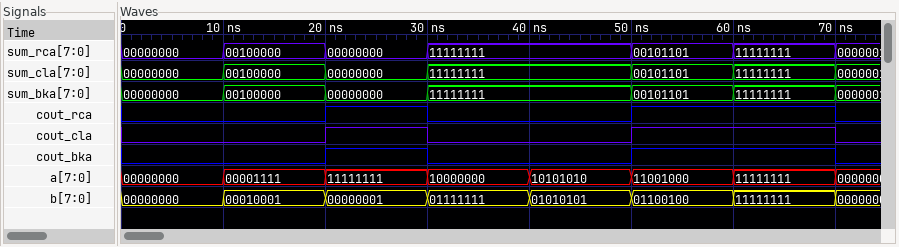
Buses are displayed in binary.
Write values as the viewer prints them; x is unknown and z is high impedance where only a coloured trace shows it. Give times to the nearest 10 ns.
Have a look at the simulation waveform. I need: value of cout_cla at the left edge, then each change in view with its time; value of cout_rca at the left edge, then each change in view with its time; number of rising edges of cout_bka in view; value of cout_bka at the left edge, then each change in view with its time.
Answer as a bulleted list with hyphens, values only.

- 0, 1 at 20 ns, 0 at 30 ns, 1 at 50 ns, 0 at 70 ns
- 0, 1 at 20 ns, 0 at 30 ns, 1 at 50 ns, 0 at 70 ns
- 2
- 0, 1 at 20 ns, 0 at 30 ns, 1 at 50 ns, 0 at 70 ns
